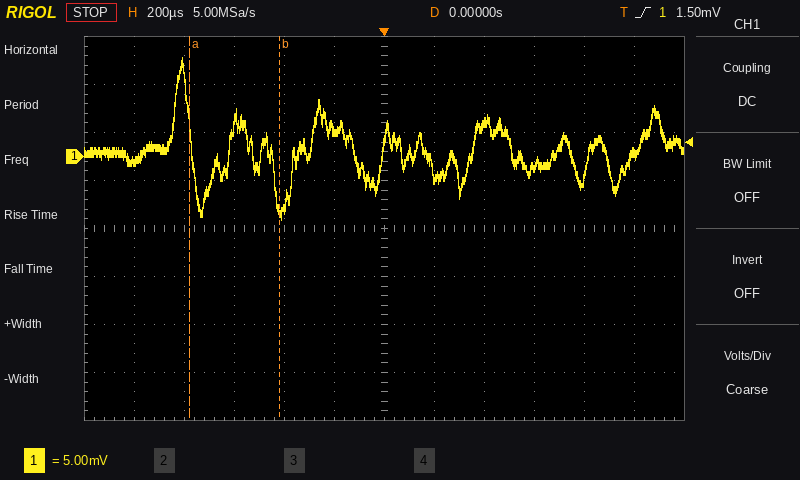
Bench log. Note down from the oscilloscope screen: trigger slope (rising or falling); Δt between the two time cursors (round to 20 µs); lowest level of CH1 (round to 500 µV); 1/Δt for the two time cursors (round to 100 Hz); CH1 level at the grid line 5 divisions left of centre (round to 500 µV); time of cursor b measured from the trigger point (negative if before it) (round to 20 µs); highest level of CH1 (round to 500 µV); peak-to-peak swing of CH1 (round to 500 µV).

rising
360 µs
-6.5 mV
2.8 kHz
-500 µV
-420 µs
10.5 mV
17.0 mV
